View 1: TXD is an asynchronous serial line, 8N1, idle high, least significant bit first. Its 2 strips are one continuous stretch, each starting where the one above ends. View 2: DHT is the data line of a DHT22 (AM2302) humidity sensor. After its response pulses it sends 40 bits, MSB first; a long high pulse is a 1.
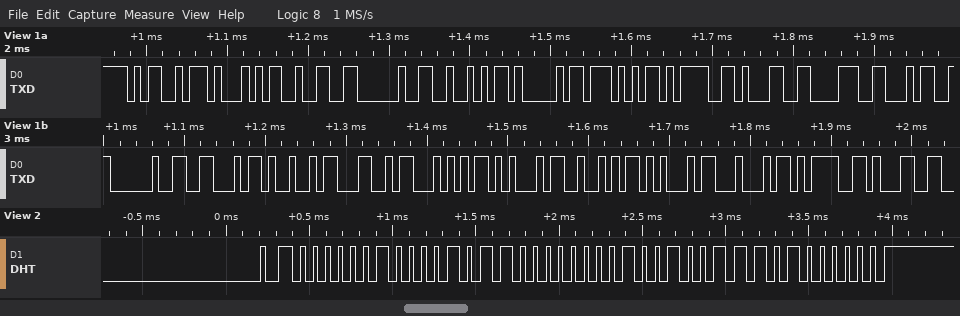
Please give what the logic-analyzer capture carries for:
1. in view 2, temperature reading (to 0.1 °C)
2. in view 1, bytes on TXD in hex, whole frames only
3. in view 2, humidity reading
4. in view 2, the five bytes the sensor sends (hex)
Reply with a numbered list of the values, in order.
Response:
1. 29.5 °C
2. 4D 51 32 20 52 41 57 3D 31 38 34 20 46 49 4C 54 45 52 45 44 3D 31
3. 53.4 %
4. 02 16 01 27 40
